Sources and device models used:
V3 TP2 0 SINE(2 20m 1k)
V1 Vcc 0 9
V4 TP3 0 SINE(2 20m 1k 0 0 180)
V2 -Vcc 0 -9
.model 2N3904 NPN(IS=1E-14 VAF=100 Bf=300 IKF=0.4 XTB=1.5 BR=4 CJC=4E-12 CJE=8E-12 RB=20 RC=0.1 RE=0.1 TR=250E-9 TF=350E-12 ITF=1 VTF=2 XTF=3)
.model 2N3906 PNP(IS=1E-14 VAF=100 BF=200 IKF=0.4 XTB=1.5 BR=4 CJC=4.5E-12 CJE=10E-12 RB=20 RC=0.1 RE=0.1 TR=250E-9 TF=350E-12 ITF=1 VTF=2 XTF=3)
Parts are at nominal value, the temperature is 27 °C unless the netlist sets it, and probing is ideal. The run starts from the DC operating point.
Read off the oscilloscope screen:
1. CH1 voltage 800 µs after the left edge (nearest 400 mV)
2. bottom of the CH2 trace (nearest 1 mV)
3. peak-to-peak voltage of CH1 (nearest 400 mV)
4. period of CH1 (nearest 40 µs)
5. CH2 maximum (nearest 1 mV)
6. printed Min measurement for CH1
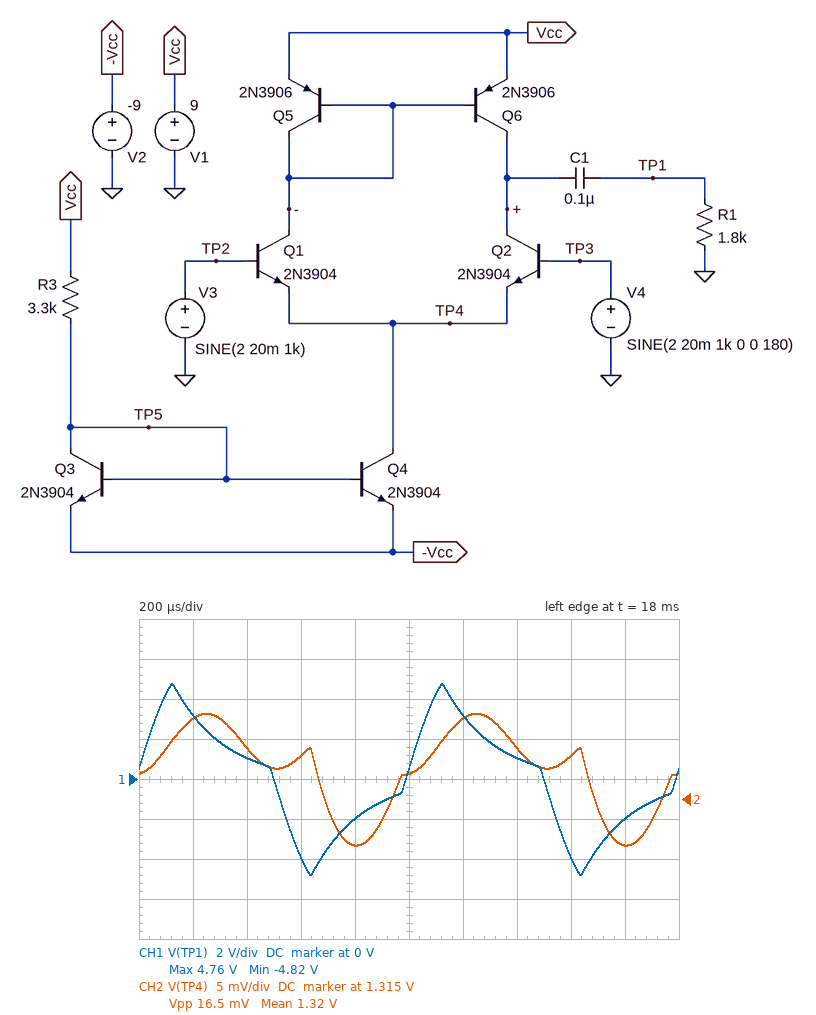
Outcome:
-2.0 V
1.309 V
9.6 V
1.00 ms
1.326 V
-4.82 V
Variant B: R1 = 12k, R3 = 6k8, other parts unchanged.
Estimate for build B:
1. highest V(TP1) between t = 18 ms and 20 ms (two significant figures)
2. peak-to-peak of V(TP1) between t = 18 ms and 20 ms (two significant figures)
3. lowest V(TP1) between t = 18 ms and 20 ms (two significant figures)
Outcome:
4.3 V
8.8 V
-4.5 V
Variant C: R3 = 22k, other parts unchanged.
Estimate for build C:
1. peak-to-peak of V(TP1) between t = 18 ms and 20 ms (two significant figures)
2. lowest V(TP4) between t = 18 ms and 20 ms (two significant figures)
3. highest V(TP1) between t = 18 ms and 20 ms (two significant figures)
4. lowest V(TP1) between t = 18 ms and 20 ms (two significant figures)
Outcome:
2.0 V
1.4 V
980 mV
-990 mV
